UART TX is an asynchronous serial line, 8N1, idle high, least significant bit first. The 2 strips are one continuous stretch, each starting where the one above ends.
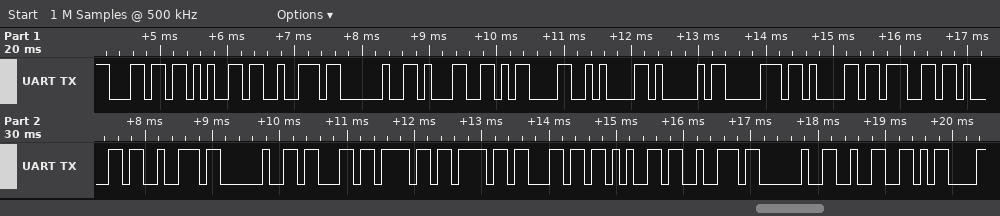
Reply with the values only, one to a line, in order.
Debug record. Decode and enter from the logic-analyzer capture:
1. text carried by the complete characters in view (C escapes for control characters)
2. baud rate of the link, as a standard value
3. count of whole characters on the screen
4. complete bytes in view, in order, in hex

"ler 1\r\nApagar cooler 2\r"
9600 baud
23
6C 65 72 20 31 0D 0A 41 70 61 67 61 72 20 63 6F 6F 6C 65 72 20 32 0D
